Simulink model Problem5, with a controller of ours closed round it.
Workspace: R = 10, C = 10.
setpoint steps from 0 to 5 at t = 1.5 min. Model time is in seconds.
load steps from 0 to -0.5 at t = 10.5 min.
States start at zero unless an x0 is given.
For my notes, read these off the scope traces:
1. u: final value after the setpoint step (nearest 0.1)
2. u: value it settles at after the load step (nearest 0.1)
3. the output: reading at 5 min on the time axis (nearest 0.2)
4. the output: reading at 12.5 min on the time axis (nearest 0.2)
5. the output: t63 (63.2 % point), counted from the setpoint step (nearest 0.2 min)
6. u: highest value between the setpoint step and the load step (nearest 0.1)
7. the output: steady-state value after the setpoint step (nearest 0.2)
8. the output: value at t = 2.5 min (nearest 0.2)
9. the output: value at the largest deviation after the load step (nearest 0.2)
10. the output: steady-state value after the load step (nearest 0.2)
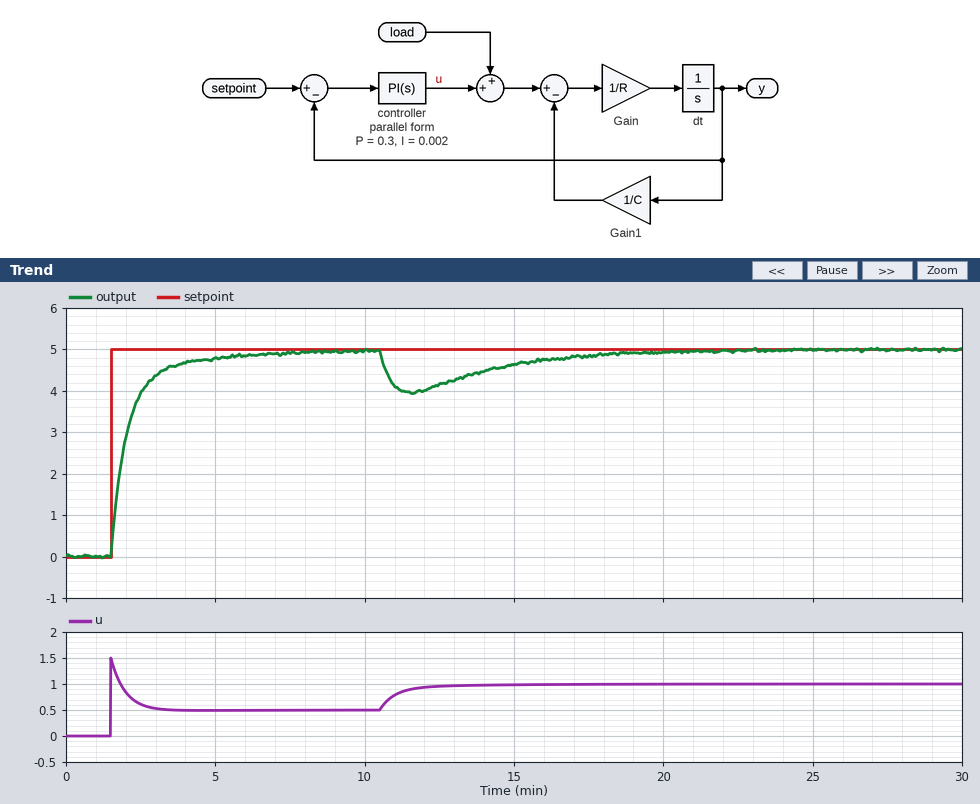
0.5
1.0
4.8
4.2
0.6 min
1.5
5.0
4.0
4.0
5.0
